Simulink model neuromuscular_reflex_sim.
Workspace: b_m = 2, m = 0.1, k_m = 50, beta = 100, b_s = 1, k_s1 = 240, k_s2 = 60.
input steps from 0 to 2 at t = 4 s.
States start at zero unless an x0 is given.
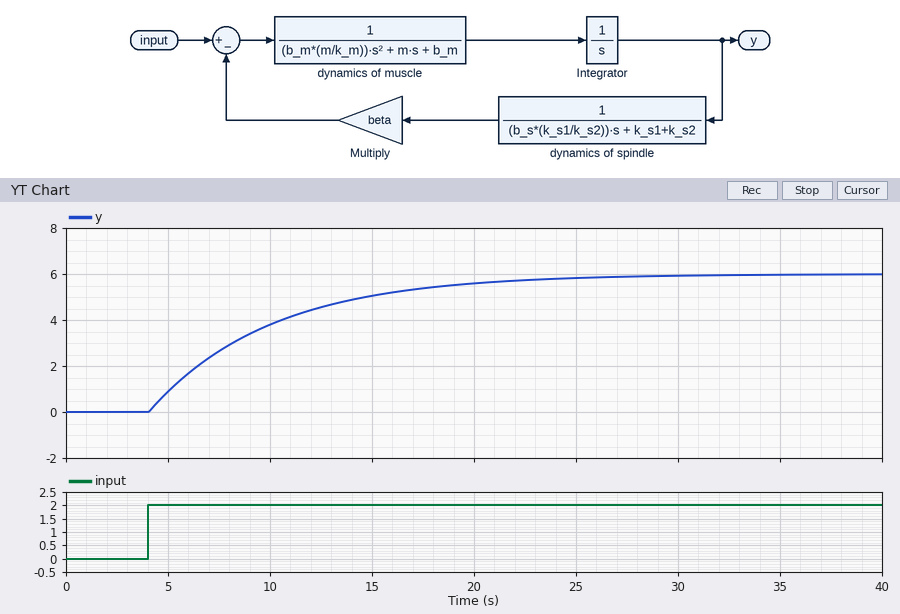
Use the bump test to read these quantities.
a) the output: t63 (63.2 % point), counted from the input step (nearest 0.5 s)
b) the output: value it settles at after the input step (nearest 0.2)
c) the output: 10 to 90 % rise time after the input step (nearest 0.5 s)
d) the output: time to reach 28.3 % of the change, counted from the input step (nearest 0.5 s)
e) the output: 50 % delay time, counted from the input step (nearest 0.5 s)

6.0 s
6.0
13.0 s
2.0 s
4.0 s
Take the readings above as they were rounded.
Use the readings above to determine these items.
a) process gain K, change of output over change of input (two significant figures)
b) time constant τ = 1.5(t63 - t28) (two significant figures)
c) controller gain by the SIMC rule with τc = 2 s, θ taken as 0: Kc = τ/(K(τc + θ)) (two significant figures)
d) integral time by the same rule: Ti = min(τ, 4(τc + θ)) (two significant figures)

3.0
6.0 s
1.0
6.0 s
